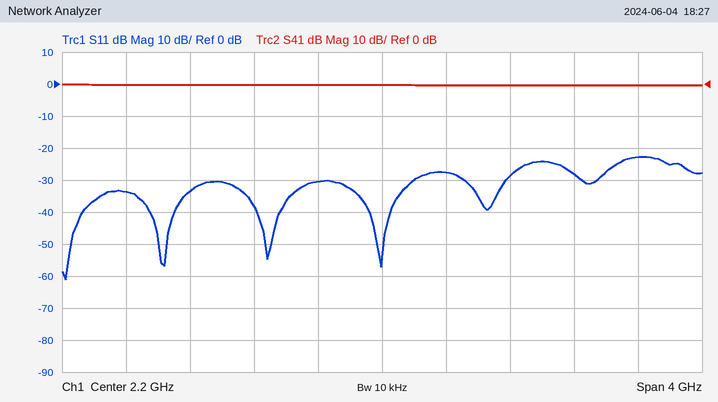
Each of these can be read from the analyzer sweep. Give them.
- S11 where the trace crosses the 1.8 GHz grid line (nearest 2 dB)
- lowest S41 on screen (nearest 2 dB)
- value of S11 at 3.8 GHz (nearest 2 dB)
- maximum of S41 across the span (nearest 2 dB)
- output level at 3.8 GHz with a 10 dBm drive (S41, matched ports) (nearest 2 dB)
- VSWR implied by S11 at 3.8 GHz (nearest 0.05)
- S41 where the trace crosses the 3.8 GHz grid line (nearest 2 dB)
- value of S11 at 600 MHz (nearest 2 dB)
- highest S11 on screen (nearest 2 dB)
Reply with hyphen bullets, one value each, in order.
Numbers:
- -30 dB
- 0 dB
- -22 dB
- 0 dB
- 10 dBm
- 1.15
- 0 dB
- -34 dB
- -22 dB
